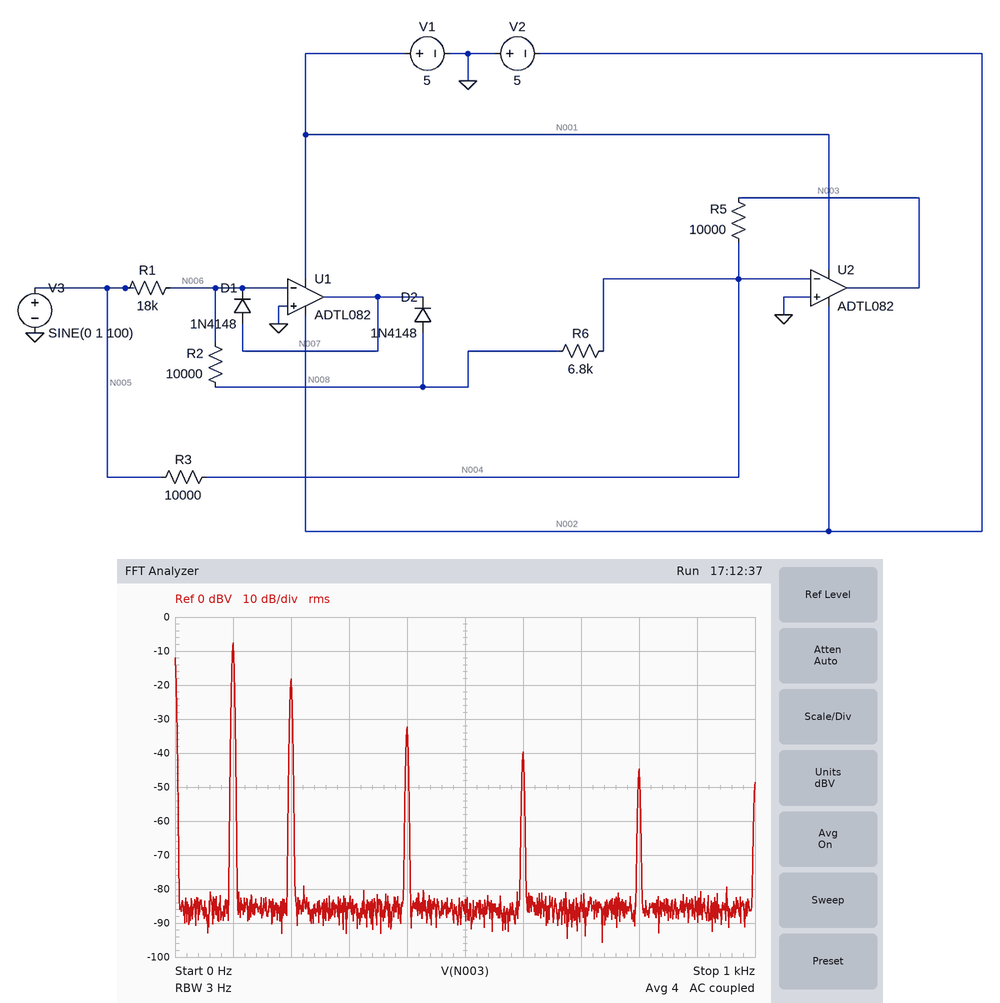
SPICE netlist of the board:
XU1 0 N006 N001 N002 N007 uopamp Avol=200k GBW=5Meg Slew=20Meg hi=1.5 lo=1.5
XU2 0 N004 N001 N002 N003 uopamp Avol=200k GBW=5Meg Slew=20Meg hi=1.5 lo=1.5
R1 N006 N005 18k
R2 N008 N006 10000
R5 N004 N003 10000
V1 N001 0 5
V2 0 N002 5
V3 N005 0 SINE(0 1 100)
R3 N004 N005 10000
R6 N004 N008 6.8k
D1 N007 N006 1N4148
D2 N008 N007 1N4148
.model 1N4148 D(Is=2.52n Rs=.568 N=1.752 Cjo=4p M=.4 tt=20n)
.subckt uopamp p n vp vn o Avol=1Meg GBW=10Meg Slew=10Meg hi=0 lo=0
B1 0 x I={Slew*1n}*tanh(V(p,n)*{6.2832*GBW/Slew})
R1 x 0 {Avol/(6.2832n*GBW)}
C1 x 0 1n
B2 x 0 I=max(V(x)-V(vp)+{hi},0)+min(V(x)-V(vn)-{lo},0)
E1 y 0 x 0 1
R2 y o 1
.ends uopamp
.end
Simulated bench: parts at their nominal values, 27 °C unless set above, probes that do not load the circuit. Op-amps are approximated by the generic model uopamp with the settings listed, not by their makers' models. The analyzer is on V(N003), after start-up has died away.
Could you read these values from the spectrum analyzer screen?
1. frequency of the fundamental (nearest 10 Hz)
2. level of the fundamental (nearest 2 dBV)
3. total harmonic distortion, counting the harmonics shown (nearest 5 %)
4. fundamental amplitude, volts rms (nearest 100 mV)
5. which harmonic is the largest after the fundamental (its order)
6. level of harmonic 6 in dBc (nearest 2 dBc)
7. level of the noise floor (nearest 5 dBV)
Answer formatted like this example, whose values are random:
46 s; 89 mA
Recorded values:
100 Hz; -8 dBV; 30 %; 400 mV; 2; -32 dBc; -85 dBV
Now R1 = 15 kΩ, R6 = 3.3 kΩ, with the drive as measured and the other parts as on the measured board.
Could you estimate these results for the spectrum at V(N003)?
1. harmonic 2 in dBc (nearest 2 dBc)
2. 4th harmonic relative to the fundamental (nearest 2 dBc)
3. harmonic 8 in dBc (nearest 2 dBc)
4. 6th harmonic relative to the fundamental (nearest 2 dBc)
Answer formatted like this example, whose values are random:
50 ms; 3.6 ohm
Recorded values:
32 dBc; 18 dBc; 6 dBc; 12 dBc
